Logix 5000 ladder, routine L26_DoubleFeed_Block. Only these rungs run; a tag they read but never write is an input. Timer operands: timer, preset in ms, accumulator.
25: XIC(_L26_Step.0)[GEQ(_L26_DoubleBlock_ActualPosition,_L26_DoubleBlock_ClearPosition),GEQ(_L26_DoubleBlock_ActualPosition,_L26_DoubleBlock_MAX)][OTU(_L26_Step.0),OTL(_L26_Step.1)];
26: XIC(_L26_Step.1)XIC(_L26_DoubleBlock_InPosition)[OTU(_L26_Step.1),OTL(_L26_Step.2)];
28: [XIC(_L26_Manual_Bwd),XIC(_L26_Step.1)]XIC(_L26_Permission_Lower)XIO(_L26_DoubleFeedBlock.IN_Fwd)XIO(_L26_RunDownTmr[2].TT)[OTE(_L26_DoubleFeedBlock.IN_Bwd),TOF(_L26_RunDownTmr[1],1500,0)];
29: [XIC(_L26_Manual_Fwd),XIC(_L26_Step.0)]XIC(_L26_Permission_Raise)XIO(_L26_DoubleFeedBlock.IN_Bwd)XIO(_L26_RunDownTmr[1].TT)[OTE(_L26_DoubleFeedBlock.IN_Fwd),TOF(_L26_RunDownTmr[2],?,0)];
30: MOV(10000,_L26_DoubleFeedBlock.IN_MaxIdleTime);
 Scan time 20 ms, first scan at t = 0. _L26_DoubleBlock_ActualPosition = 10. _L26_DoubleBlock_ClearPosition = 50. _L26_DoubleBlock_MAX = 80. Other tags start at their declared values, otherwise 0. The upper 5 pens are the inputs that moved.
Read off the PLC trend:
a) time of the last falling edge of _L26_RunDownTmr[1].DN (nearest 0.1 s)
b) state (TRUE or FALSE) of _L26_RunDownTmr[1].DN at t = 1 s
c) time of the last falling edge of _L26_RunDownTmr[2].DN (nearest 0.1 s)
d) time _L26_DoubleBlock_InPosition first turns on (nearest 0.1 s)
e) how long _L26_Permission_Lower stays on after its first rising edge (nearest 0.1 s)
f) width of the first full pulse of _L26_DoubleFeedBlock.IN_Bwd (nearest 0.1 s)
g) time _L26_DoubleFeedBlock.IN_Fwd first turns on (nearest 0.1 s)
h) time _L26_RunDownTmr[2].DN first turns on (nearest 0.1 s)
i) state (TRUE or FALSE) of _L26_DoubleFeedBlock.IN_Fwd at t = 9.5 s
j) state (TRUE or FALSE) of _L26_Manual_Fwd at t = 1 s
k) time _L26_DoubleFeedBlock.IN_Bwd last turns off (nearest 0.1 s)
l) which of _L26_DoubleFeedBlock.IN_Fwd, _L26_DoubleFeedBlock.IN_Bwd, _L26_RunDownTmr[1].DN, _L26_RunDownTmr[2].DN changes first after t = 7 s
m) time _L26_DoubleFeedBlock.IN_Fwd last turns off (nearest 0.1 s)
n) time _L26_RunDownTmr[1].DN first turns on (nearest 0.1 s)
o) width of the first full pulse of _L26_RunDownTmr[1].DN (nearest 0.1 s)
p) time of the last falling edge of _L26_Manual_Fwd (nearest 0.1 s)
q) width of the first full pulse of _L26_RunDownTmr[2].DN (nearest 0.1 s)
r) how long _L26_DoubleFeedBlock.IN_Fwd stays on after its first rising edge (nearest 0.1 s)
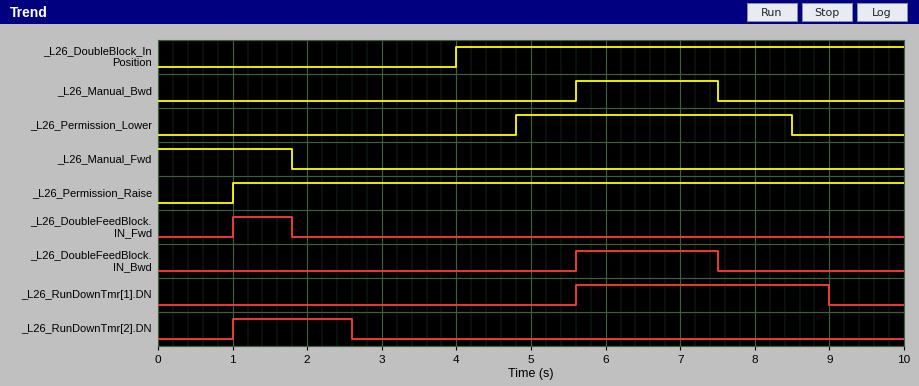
9.0 s
FALSE
2.6 s
4.0 s
3.7 s
1.9 s
1.0 s
1.0 s
FALSE
TRUE
7.5 s
_L26_DoubleFeedBlock.IN_Bwd
1.8 s
5.6 s
3.4 s
1.8 s
1.6 s
0.8 s
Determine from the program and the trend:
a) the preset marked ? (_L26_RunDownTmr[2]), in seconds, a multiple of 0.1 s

0.8 s
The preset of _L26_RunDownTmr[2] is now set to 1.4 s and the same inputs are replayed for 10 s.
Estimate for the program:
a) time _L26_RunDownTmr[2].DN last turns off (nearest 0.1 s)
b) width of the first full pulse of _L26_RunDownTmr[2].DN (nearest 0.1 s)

3.2 s
2.2 s
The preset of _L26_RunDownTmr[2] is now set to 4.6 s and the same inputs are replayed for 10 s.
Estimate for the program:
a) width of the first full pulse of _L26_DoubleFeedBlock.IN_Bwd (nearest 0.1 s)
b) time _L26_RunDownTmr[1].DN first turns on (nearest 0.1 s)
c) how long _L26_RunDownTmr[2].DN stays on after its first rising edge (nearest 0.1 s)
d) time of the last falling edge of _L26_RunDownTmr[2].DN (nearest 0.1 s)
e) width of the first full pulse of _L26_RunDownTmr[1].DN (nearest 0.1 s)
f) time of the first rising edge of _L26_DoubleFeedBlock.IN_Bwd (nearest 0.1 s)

1.1 s
6.4 s
5.4 s
6.4 s
2.6 s
6.4 s
